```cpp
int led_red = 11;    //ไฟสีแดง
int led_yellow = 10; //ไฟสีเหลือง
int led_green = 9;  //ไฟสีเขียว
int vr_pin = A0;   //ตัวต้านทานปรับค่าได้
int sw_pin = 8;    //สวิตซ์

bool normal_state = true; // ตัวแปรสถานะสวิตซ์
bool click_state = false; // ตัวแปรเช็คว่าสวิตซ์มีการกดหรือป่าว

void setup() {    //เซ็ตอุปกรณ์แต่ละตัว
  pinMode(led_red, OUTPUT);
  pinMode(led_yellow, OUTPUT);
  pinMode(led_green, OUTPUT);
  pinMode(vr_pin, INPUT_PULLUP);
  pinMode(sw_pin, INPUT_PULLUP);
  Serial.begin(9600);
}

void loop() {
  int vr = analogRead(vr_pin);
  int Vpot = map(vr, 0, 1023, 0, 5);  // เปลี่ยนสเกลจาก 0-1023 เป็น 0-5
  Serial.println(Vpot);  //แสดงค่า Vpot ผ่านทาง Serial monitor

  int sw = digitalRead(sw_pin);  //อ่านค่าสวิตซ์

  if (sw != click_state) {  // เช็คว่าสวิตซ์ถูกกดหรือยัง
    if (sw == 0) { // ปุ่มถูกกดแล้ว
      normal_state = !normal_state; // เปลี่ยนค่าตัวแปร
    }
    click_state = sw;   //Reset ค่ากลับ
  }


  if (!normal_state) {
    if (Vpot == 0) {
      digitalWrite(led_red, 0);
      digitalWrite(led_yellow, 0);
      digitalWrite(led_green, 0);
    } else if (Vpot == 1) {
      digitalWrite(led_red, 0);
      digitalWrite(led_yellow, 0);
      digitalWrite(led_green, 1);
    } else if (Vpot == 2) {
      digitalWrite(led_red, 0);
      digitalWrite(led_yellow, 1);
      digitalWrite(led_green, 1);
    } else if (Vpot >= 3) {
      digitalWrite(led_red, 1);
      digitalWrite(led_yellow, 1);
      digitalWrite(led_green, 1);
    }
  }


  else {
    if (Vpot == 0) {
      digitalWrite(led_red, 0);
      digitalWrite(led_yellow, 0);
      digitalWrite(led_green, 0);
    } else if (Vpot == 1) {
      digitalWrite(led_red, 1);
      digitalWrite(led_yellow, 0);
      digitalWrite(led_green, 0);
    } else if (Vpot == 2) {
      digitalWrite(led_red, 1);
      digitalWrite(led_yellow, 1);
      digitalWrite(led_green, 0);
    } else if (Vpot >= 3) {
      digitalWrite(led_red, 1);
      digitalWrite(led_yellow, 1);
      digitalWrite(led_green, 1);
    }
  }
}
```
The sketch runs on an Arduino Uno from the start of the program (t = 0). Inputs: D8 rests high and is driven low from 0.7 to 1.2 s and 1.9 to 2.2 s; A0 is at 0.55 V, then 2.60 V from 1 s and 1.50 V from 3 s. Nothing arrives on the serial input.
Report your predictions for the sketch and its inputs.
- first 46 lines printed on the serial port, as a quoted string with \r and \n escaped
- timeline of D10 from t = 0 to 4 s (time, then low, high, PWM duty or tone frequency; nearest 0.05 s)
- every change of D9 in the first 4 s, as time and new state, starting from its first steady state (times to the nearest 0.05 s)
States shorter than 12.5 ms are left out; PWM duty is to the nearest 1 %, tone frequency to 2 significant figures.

"0\r\n0\r\n0\r\n0\r\n0\r\n0\r\n0\r\n0\r\n0\r\n0\r\n0\r\n0\r\n0\r\n0\r\n0\r\n0\r\n0\r\n0\r\n0\r\n0\r\n0\r\n0\r\n0\r\n0\r\n0\r\n0\r\n0\r\n0\r\n0\r\n0\r\n0\r\n0\r\n0\r\n0\r\n0\r\n0\r\n0\r\n0\r\n0\r\n0\r\n0\r\n0\r\n0\r\n0\r\n0\r\n0\r\n"
0 s low; 1 s high; 3 s low
0 s low; 1 s high; 1.9 s low
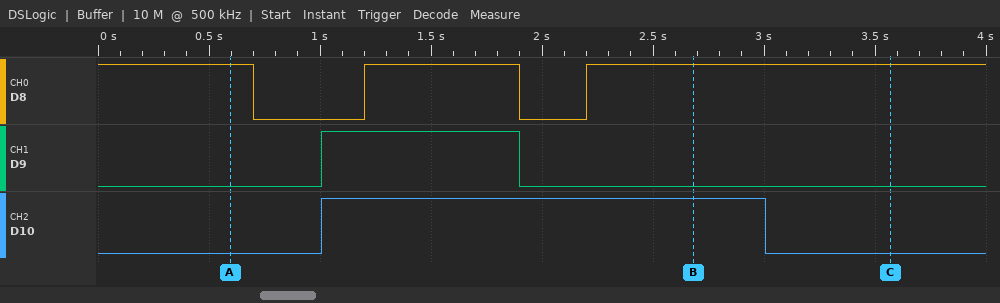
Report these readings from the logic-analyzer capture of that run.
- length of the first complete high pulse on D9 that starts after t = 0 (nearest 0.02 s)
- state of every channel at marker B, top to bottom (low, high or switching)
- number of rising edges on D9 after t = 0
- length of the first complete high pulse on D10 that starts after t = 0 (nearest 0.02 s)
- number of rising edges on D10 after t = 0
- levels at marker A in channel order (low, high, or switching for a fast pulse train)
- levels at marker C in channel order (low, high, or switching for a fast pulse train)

0.90 s
D8 high, D9 low, D10 high
1
2.00 s
1
D8 high, D9 low, D10 low
D8 high, D9 low, D10 low
